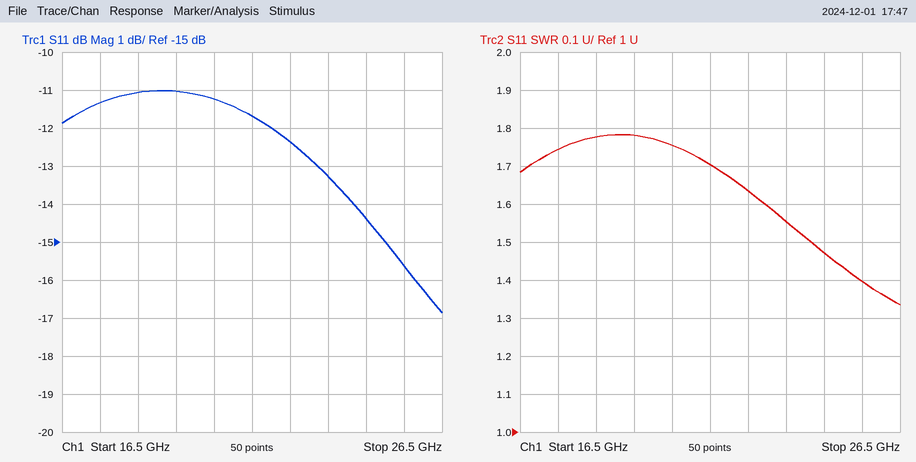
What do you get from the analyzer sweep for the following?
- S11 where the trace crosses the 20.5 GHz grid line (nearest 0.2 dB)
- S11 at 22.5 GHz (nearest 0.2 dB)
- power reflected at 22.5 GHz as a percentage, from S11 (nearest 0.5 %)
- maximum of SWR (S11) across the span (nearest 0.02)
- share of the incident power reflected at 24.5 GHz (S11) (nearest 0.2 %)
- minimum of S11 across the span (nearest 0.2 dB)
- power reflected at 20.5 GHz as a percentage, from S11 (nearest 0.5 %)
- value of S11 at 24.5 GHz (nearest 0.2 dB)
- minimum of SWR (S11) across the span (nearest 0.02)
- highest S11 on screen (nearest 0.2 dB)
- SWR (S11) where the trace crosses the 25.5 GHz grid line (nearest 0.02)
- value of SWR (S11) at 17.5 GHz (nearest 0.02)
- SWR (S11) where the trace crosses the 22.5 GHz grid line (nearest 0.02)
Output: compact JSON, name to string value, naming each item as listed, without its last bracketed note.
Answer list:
{"S11 where the trace crosses the 20.5 GHz grid line": "-11.2 dB", "S11 at 22.5 GHz": "-12.4 dB", "power reflected at 22.5 GHz as a percentage, from S11": "6.0 %", "maximum of SWR (S11) across the span": "1.78", "share of the incident power reflected at 24.5 GHz (S11)": "3.6 %", "minimum of S11 across the span": "-16.8 dB", "power reflected at 20.5 GHz as a percentage, from S11": "7.5 %", "value of S11 at 24.5 GHz": "-14.4 dB", "minimum of SWR (S11) across the span": "1.34", "highest S11 on screen": "-11.0 dB", "SWR (S11) where the trace crosses the 25.5 GHz grid line": "1.40", "value of SWR (S11) at 17.5 GHz": "1.74", "SWR (S11) where the trace crosses the 22.5 GHz grid line": "1.64"}
